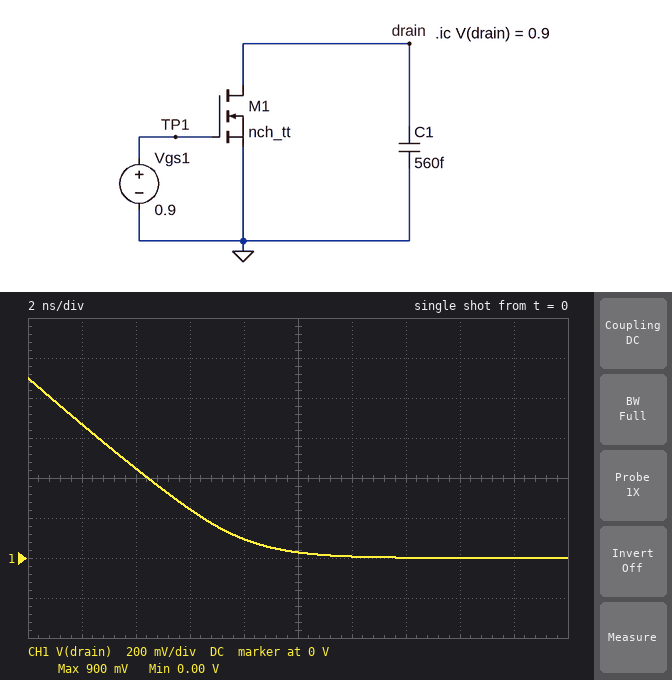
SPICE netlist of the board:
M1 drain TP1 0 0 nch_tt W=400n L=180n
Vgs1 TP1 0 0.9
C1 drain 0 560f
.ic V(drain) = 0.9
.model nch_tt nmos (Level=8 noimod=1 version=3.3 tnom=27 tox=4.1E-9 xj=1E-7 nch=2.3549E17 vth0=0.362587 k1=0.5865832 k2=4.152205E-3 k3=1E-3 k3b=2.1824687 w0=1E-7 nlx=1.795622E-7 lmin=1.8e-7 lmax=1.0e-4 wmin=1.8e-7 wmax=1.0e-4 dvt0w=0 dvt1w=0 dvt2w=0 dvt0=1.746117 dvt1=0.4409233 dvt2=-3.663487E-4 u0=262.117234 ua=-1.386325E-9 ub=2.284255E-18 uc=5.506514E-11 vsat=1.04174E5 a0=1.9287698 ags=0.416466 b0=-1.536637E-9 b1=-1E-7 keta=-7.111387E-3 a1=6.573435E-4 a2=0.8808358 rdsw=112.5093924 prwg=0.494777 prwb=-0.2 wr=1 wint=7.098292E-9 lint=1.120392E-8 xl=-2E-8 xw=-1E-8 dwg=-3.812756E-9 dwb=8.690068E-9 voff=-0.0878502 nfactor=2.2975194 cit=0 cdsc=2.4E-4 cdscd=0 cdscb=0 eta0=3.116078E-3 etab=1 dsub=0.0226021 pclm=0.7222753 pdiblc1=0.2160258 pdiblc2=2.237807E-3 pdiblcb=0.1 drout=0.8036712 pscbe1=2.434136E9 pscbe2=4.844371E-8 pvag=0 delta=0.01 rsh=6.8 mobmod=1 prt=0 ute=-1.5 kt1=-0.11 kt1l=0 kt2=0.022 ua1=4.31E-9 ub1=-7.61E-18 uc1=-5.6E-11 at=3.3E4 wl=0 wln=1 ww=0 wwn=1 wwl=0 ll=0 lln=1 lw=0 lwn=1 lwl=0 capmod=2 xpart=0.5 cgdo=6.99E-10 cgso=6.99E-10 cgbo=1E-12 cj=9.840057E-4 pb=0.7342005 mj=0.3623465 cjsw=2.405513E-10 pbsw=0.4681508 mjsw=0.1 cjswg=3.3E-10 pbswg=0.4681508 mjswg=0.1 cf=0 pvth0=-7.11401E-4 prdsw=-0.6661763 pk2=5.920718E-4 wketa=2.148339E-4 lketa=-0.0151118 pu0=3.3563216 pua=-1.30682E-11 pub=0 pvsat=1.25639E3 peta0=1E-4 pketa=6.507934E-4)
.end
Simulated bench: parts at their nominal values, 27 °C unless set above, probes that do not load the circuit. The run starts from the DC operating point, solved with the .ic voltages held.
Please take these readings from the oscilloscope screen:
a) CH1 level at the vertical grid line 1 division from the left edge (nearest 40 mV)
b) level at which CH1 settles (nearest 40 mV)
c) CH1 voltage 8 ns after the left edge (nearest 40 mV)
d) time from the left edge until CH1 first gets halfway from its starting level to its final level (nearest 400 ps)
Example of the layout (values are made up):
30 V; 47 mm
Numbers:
680 mV; 0 V; 80 mV; 4.0 ns
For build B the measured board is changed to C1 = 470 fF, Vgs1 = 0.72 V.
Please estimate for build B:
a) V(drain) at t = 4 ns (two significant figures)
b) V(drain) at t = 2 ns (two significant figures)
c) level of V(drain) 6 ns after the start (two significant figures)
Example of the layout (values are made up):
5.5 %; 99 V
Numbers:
660 mV; 780 mV; 540 mV
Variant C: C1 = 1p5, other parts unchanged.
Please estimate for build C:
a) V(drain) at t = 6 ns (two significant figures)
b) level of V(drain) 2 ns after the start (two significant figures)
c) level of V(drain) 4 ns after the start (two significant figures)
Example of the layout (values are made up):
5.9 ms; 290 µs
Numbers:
640 mV; 810 mV; 730 mV
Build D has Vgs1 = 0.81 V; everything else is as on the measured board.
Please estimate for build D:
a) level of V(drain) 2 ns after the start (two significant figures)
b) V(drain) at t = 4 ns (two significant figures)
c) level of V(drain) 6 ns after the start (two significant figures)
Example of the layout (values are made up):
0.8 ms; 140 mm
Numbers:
730 mV; 570 mV; 420 mV
